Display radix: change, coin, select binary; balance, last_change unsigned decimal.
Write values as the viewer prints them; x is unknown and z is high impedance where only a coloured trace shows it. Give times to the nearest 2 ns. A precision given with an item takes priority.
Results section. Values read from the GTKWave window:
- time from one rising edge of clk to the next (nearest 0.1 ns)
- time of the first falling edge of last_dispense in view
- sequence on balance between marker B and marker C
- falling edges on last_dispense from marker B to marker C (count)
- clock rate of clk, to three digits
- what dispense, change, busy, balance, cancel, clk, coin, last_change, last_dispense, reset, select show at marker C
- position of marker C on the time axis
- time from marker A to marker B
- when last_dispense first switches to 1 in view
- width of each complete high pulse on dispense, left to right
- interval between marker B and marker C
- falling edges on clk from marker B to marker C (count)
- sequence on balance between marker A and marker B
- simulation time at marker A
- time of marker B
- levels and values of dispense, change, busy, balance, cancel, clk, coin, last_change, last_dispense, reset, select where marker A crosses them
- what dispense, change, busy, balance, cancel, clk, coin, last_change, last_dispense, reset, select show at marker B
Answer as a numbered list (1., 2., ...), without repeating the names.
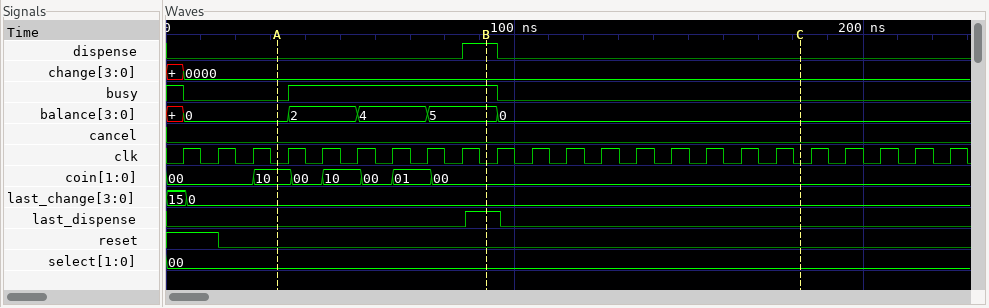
1. 10 ns
2. 96 ns
3. 5, 0
4. 1
5. 100 MHz
6. dispense=0, change=0000, busy=0, balance=0, cancel=0, clk=0, coin=00, last_change=0, last_dispense=0, reset=0, select=00
7. 182 ns
8. 60 ns
9. 86 ns
10. 10 ns
11. 90 ns
12. 9
13. 0, 2, 4, 5
14. 32 ns
15. 92 ns
16. dispense=0, change=0000, busy=0, balance=0, cancel=0, clk=0, coin=10, last_change=0, last_dispense=0, reset=0, select=00
17. dispense=1, change=0000, busy=1, balance=5, cancel=0, clk=0, coin=00, last_change=0, last_dispense=1, reset=0, select=00
